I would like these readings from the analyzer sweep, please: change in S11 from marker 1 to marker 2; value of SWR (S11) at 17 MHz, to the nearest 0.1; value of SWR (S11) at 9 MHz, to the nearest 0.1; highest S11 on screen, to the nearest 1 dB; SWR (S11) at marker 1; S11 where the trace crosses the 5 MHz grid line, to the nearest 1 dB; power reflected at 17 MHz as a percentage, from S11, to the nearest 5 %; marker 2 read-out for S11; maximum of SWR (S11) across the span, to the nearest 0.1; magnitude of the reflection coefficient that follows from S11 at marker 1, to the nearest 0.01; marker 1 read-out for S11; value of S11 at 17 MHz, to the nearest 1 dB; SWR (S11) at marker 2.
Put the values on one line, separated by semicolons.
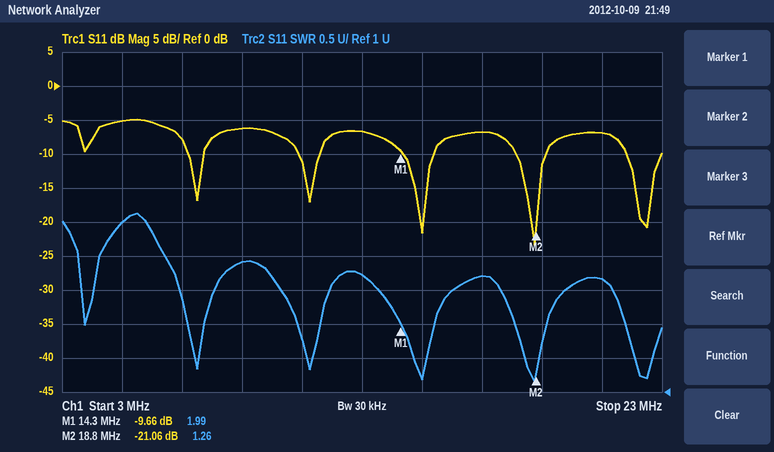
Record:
-11.40 dB; 2.7; 2.9; -5 dB; 1.99; -5 dB; 20 %; -21.06 dB; 3.6; 0.33; -9.66 dB; -7 dB; 1.26
